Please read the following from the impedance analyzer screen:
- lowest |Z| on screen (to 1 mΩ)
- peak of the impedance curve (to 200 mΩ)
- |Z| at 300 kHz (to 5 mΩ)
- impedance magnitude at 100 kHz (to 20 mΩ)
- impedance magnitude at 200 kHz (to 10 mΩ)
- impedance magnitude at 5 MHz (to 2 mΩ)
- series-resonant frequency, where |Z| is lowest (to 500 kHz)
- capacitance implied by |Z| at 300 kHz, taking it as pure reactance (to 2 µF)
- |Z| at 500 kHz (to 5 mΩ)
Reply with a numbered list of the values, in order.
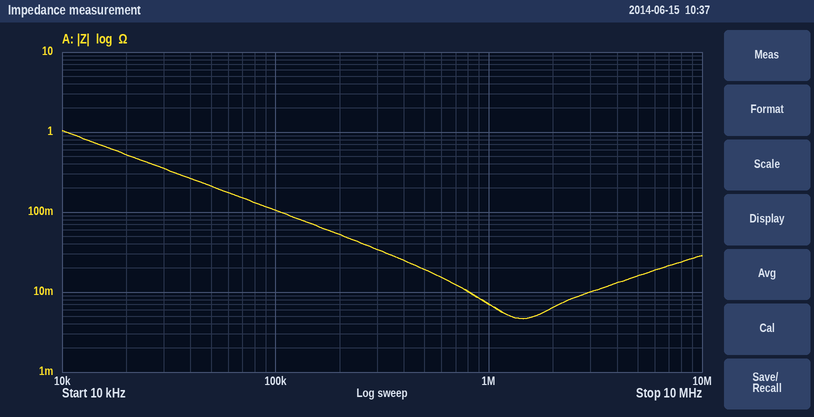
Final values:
1. 5 mΩ
2. 1.0 Ω
3. 35 mΩ
4. 100 mΩ
5. 50 mΩ
6. 16 mΩ
7. 1.5 MHz
8. 16 µF
9. 20 mΩ
